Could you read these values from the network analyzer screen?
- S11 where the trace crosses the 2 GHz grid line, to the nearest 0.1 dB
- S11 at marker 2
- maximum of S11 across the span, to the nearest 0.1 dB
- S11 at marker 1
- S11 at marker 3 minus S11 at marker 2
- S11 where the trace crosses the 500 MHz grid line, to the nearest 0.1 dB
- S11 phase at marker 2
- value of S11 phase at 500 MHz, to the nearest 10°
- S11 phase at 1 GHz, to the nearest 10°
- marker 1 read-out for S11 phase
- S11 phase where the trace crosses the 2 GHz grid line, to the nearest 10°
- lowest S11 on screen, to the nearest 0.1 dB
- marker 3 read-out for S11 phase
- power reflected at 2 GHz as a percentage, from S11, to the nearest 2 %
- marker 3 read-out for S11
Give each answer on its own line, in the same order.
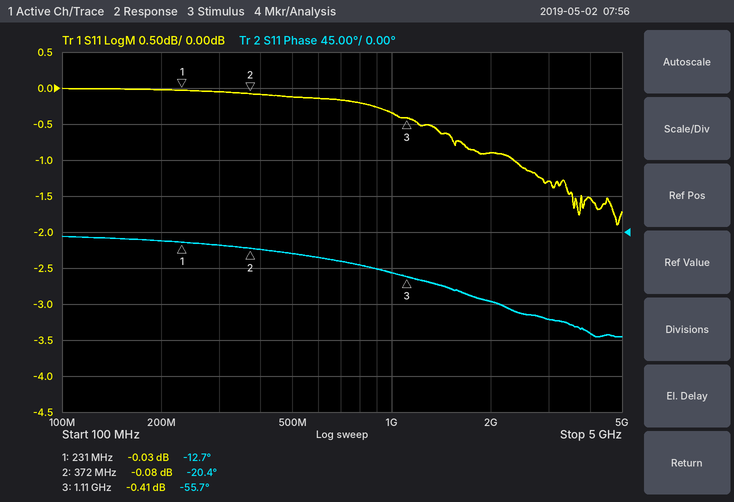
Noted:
-0.9 dB
-0.08 dB
0.0 dB
-0.03 dB
-0.33 dB
-0.1 dB
-20.4°
-30°
-50°
-12.7°
-90°
-1.9 dB
-55.7°
82 %
-0.41 dB
